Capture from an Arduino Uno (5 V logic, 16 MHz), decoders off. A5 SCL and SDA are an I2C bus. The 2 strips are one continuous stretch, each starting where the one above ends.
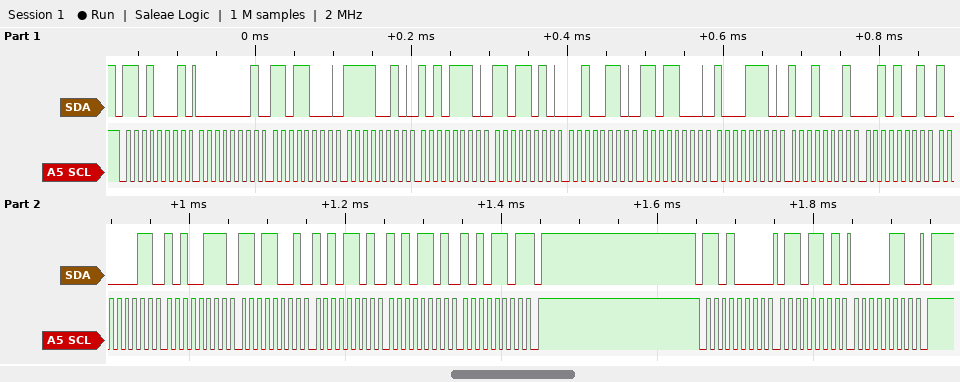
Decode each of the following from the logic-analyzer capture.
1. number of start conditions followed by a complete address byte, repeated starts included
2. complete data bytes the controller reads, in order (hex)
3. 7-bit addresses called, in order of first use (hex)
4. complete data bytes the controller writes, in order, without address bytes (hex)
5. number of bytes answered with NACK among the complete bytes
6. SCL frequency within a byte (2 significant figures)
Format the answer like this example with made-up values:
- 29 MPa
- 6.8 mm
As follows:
- 2
- 01 D8 F2 AE DA 26 D8 8E 91 29 83 A7 D9 AD AD AD
- 0x68
- 6D 06
- 1
- 100 kHz
